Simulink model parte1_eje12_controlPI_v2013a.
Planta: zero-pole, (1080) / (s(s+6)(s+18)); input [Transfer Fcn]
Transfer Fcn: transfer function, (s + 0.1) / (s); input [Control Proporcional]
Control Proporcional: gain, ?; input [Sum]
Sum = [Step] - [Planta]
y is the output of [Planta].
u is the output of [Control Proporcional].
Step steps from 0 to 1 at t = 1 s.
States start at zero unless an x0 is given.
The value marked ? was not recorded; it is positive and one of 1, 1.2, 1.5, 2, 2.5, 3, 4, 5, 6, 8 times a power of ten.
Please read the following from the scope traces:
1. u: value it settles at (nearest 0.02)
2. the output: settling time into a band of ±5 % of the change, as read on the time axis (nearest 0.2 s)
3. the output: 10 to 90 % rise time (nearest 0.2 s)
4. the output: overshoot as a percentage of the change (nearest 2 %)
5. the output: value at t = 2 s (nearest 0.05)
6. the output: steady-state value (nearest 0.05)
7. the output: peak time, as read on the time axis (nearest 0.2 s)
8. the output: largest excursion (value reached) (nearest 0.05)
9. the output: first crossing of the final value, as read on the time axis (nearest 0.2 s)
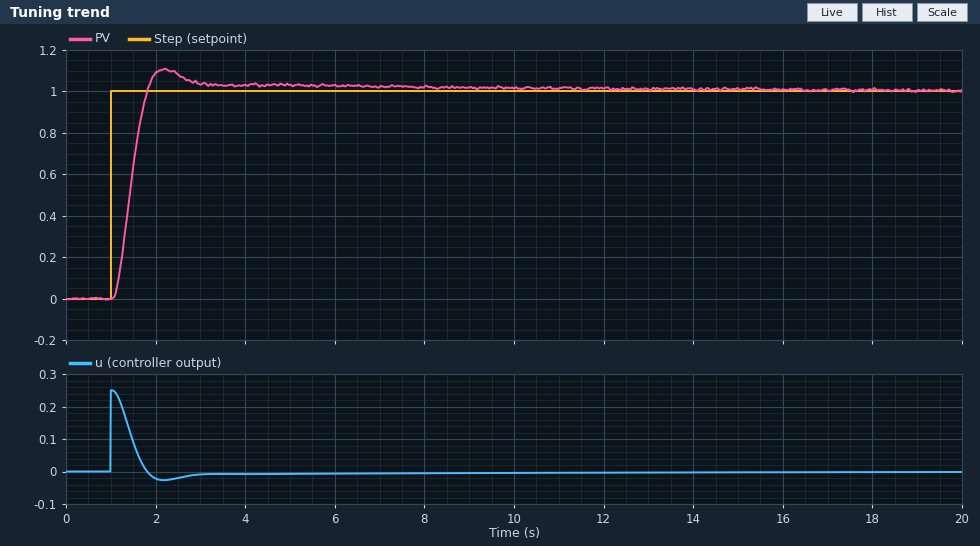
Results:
0.00
2.8 s
0.6 s
10 %
1.10
1.00
2.2 s
1.10
1.8 s
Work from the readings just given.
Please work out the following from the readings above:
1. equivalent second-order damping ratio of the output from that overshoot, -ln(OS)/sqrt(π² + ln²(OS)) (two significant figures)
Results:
0.59
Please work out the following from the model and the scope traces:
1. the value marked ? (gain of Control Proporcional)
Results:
0.25
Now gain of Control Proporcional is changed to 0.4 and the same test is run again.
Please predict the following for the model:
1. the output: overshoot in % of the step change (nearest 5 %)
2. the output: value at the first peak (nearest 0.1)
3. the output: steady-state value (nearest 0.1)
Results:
20 %
1.2
1.0
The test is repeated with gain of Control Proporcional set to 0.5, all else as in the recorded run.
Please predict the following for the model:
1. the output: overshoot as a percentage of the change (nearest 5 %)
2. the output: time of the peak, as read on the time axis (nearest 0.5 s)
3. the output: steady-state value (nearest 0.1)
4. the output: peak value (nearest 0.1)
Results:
30 %
1.5 s
1.0
1.3
